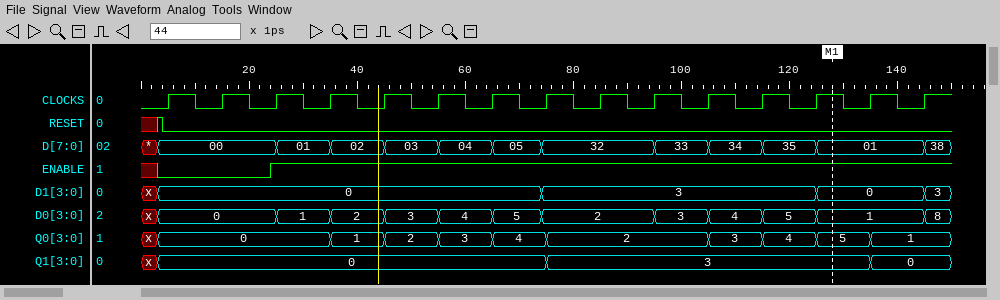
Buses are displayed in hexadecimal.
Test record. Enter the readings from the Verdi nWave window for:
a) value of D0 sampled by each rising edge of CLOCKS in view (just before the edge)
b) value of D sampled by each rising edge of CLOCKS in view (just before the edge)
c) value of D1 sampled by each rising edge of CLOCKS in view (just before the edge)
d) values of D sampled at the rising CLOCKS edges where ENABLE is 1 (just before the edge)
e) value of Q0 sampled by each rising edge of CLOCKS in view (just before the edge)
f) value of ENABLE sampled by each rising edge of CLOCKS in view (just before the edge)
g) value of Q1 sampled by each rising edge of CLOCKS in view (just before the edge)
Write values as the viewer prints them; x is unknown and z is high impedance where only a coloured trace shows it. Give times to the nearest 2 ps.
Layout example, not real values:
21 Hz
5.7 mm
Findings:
0, 0, 0, 1, 2, 3, 4, 2, 2, 2, 3, 4, 5, 1, 1
00, 00, 00, 01, 02, 03, 04, 32, 32, 32, 33, 34, 35, 01, 01
0, 0, 0, 0, 0, 0, 0, 3, 3, 3, 3, 3, 3, 0, 0
00, 01, 02, 03, 04, 32, 32, 32, 33, 34, 35, 01, 01
0, 0, 0, 0, 1, 2, 3, 4, 2, 2, 2, 3, 4, 5, 1
0 0 1 1 1 1 1 1 1 1 1 1 1 1 1
0, 0, 0, 0, 0, 0, 0, 0, 3, 3, 3, 3, 3, 3, 0
